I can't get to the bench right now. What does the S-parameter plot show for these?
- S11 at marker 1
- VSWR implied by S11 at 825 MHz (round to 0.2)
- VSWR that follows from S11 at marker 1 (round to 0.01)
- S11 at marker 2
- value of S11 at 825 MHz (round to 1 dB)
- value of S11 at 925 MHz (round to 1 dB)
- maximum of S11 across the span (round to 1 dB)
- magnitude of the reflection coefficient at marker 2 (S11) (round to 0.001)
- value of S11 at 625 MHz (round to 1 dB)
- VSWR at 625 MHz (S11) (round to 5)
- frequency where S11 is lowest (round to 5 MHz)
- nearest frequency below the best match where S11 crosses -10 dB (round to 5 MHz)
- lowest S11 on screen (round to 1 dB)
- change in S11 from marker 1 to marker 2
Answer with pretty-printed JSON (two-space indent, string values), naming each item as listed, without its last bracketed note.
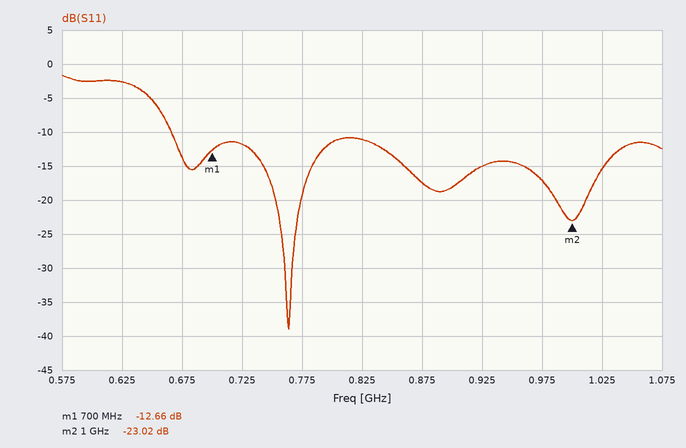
{
  "S11 at marker 1": "-12.66 dB",
  "VSWR implied by S11 at 825 MHz": "1.8",
  "VSWR that follows from S11 at marker 1": "1.61",
  "S11 at marker 2": "-23.02 dB",
  "value of S11 at 825 MHz": "-11 dB",
  "value of S11 at 925 MHz": "-15 dB",
  "maximum of S11 across the span": "-2 dB",
  "magnitude of the reflection coefficient at marker 2 (S11)": "0.071",
  "value of S11 at 625 MHz": "-3 dB",
  "VSWR at 625 MHz (S11)": "5",
  "frequency where S11 is lowest": "765 MHz",
  "nearest frequency below the best match where S11 crosses -10 dB": "665 MHz",
  "lowest S11 on screen": "-39 dB",
  "change in S11 from marker 1 to marker 2": "-10.36 dB"
}
